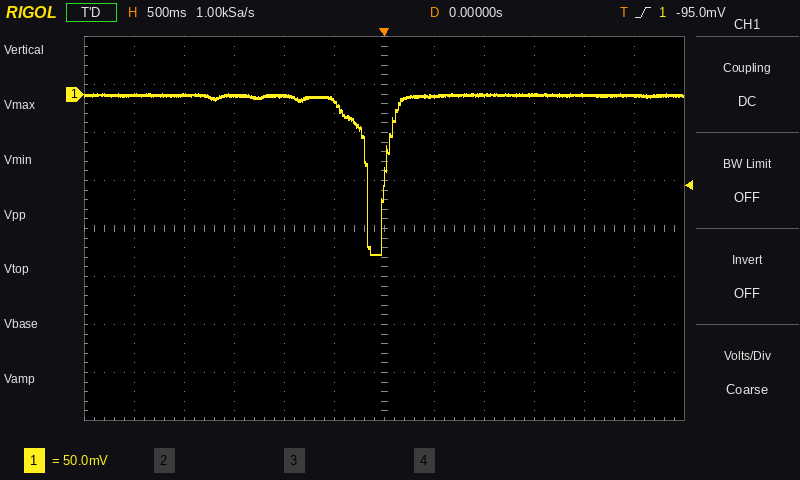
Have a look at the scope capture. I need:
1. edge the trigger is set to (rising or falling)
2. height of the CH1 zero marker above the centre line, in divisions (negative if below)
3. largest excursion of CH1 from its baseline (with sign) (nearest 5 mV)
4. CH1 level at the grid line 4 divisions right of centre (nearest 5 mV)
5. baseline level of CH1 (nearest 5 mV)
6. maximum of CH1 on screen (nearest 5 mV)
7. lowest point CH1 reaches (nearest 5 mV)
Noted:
rising
+2.8 div
-165 mV
0 mV
0 mV
0 mV
-165 mV
